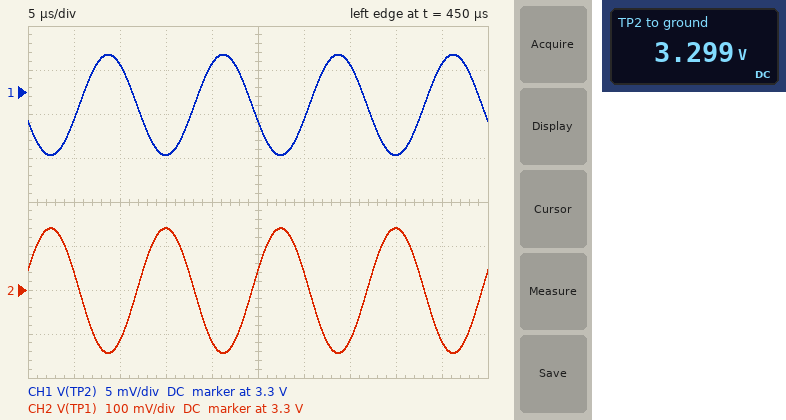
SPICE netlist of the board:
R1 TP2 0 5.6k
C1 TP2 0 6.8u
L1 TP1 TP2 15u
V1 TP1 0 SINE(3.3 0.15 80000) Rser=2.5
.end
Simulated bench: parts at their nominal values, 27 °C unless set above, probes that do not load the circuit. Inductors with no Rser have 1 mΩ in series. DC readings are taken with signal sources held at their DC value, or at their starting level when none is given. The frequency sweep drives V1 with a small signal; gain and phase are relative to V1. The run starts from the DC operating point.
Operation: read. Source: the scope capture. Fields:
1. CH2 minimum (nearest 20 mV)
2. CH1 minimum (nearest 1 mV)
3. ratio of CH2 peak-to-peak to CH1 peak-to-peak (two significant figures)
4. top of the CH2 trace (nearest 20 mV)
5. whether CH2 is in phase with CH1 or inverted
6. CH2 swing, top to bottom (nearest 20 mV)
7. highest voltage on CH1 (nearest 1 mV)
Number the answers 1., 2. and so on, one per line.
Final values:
1. 3.16 V
2. 3.293 V
3. 25
4. 3.44 V
5. inverted
6. 280 mV
7. 3.304 V
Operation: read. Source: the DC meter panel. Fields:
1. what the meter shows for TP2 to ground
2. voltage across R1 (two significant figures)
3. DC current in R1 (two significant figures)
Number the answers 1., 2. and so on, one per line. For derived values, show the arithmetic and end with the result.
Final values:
1. 3.299 V
2. 3.299 V = 3.3 V
3. (3.299 V) / 5.6 kΩ = 590 µA
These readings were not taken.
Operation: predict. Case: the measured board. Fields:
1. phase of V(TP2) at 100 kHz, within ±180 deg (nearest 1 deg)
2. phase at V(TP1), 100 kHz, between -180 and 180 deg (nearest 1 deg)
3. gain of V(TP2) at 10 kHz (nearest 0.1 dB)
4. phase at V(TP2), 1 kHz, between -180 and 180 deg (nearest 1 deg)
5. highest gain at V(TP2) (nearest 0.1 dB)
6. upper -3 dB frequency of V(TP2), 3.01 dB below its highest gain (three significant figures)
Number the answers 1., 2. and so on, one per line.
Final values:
1. -165 deg
2. 15 deg
3. -1.8 dB
4. -6 deg
5. 0 dB
6. 12.9 kHz
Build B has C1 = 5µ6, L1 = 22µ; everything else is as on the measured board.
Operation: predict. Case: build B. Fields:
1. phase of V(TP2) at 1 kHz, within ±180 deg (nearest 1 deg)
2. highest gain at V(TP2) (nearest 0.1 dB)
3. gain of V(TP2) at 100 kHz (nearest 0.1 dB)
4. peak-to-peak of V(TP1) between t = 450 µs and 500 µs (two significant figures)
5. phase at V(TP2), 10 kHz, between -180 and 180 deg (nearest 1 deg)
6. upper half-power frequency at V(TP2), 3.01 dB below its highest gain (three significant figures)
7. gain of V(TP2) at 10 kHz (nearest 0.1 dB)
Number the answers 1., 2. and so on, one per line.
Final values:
1. -5 deg
2. 0.2 dB
3. -33.7 dB
4. 290 mV
5. -60 deg
6. 15.6 kHz
7. -0.2 dB
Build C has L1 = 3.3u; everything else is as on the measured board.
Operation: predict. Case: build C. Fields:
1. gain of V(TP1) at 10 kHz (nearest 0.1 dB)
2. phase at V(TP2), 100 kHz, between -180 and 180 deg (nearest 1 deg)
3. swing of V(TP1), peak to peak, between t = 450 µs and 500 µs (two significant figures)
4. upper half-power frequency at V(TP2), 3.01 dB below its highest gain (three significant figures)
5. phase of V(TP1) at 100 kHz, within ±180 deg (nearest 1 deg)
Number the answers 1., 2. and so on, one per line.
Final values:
1. -3.8 dB
2. -126 deg
3. 140 mV
4. 10.1 kHz
5. 54 deg
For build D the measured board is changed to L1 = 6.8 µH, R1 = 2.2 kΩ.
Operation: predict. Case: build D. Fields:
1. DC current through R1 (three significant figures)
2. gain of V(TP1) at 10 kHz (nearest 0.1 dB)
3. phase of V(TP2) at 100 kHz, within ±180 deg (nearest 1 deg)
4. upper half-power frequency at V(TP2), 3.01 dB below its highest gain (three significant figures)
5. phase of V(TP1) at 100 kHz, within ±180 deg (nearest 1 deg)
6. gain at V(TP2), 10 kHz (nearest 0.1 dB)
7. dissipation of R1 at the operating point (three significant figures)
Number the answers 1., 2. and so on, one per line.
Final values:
1. 1.50 mA
2. -4.3 dB
3. -148 deg
4. 11.1 kHz
5. 32 deg
6. -2.6 dB
7. 4.94 mW
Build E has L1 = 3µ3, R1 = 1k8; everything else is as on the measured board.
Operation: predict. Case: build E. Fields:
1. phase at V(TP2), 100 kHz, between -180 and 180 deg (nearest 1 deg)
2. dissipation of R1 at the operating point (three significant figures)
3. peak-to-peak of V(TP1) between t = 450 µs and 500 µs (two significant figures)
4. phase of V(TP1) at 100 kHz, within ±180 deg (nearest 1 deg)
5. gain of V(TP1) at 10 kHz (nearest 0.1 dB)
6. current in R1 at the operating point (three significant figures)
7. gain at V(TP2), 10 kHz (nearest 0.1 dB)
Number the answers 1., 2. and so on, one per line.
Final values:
1. -126 deg
2. 6.03 mW
3. 140 mV
4. 54 deg
5. -3.8 dB
6. 1.83 mA
7. -3.0 dB
